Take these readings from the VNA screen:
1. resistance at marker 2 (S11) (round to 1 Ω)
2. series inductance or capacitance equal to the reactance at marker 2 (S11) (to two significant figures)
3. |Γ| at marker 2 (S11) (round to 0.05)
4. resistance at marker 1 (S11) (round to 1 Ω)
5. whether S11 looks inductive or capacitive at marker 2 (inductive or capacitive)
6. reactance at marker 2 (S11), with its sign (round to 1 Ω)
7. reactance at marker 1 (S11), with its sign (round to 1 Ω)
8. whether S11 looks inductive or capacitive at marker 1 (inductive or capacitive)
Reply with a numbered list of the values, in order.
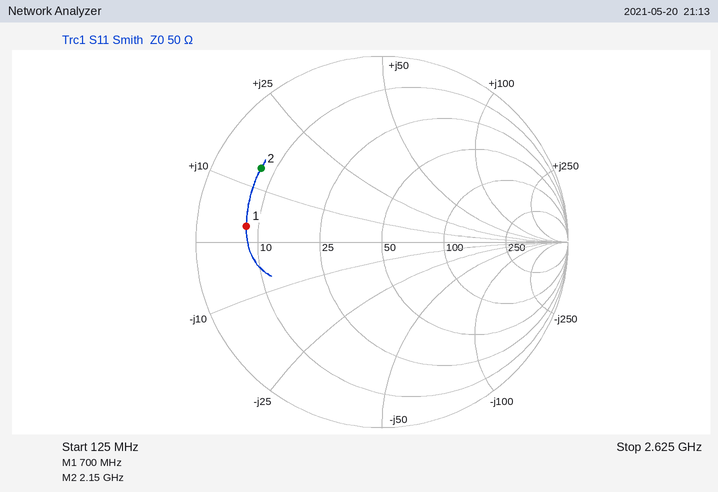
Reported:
1. 7 Ω
2. 1.0 nH
3. 0.75
4. 8 Ω
5. inductive
6. +14 Ω
7. +3 Ω
8. inductive
